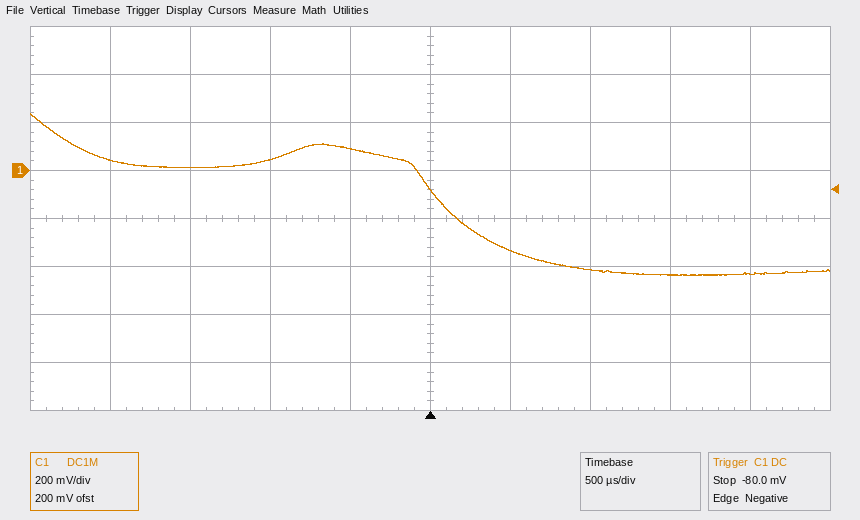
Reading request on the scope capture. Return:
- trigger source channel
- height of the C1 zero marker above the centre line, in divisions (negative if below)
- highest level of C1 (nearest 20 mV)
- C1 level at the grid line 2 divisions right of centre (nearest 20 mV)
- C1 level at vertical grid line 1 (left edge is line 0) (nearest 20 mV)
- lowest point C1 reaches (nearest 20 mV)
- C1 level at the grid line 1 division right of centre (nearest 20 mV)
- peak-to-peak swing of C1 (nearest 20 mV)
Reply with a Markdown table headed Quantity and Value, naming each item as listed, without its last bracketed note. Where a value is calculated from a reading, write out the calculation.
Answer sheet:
| Quantity | Value |
|---|---|
| trigger source channel | C1 |
| height of the C1 zero marker above the centre line, in divisions | +1.0 div |
| highest level of C1 | 240 mV |
| C1 level at the grid line 2 divisions right of centre | -420 mV |
| C1 level at vertical grid line 1 (left edge is line 0) | 40 mV |
| lowest point C1 reaches | -440 mV |
| C1 level at the grid line 1 division right of centre | -340 mV |
| peak-to-peak swing of C1 | 240 mV − (-440 mV) = 680 mV |
